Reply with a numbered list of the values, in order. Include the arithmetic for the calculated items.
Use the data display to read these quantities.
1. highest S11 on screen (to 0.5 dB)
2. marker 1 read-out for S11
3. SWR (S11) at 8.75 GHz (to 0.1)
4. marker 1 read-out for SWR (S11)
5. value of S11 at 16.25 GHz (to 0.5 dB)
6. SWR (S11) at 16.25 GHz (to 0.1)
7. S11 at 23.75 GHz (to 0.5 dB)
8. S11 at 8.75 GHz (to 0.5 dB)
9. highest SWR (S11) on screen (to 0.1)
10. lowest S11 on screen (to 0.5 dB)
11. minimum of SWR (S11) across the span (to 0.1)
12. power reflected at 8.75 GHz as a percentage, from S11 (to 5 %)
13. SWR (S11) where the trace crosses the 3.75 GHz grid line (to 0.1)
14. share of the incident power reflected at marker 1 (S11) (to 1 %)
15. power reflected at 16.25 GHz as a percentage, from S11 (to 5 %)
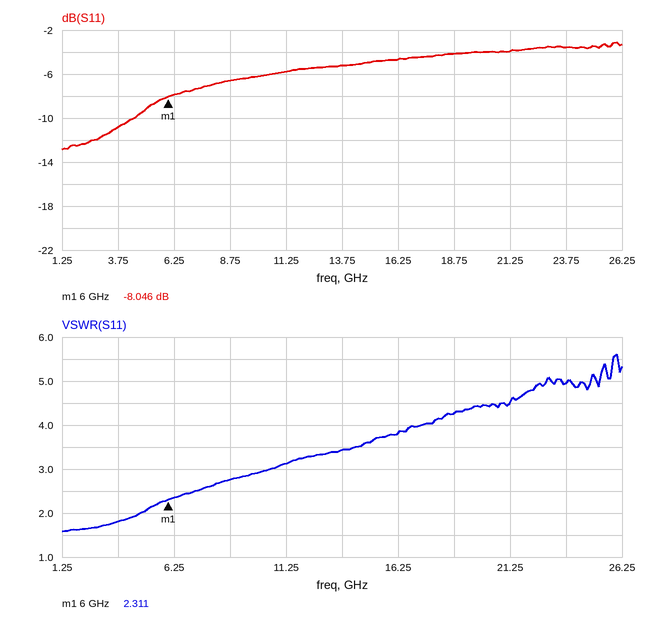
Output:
1. -3.0 dB
2. -8.046 dB
3. 2.8
4. 2.311
5. -4.5 dB
6. 3.8
7. -3.5 dB
8. -6.5 dB
9. 5.6
10. -13.0 dB
11. 1.6
12. 10^(-6.5/10) ≈ 22.4 %, so 20 % to the nearest 5 %
13. 1.8
14. 10^(-8.046/10) ≈ 16 %
15. 10^(-4.5/10) ≈ 35 %
